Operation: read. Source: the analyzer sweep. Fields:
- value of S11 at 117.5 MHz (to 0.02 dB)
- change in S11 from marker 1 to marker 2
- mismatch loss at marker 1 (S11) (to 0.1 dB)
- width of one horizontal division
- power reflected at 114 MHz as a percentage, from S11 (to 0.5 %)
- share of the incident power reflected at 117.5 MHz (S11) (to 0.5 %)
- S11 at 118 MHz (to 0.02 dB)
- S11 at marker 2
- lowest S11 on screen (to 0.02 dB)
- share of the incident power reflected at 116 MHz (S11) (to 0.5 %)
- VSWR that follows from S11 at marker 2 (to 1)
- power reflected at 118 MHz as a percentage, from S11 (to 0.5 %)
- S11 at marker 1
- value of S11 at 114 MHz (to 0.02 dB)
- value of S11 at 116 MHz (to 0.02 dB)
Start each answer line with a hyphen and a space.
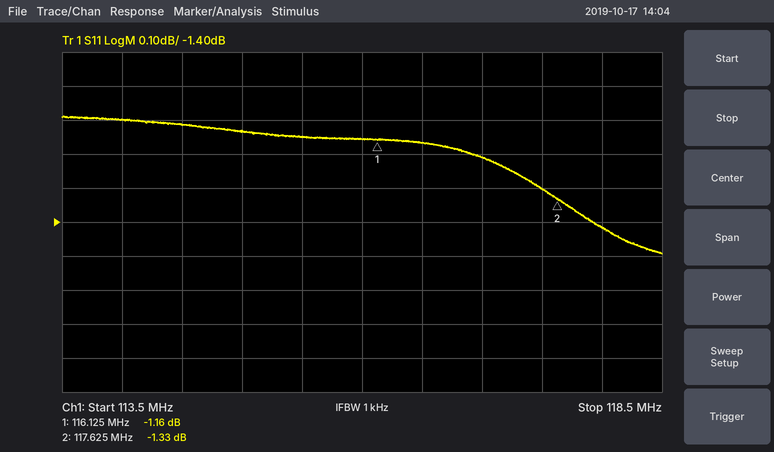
- -1.30 dB
- -0.17 dB
- 6.3 dB
- 500 kHz
- 77.5 %
- 74.0 %
- -1.42 dB
- -1.33 dB
- -1.50 dB
- 76.5 %
- 13
- 72.0 %
- -1.16 dB
- -1.10 dB
- -1.16 dB
